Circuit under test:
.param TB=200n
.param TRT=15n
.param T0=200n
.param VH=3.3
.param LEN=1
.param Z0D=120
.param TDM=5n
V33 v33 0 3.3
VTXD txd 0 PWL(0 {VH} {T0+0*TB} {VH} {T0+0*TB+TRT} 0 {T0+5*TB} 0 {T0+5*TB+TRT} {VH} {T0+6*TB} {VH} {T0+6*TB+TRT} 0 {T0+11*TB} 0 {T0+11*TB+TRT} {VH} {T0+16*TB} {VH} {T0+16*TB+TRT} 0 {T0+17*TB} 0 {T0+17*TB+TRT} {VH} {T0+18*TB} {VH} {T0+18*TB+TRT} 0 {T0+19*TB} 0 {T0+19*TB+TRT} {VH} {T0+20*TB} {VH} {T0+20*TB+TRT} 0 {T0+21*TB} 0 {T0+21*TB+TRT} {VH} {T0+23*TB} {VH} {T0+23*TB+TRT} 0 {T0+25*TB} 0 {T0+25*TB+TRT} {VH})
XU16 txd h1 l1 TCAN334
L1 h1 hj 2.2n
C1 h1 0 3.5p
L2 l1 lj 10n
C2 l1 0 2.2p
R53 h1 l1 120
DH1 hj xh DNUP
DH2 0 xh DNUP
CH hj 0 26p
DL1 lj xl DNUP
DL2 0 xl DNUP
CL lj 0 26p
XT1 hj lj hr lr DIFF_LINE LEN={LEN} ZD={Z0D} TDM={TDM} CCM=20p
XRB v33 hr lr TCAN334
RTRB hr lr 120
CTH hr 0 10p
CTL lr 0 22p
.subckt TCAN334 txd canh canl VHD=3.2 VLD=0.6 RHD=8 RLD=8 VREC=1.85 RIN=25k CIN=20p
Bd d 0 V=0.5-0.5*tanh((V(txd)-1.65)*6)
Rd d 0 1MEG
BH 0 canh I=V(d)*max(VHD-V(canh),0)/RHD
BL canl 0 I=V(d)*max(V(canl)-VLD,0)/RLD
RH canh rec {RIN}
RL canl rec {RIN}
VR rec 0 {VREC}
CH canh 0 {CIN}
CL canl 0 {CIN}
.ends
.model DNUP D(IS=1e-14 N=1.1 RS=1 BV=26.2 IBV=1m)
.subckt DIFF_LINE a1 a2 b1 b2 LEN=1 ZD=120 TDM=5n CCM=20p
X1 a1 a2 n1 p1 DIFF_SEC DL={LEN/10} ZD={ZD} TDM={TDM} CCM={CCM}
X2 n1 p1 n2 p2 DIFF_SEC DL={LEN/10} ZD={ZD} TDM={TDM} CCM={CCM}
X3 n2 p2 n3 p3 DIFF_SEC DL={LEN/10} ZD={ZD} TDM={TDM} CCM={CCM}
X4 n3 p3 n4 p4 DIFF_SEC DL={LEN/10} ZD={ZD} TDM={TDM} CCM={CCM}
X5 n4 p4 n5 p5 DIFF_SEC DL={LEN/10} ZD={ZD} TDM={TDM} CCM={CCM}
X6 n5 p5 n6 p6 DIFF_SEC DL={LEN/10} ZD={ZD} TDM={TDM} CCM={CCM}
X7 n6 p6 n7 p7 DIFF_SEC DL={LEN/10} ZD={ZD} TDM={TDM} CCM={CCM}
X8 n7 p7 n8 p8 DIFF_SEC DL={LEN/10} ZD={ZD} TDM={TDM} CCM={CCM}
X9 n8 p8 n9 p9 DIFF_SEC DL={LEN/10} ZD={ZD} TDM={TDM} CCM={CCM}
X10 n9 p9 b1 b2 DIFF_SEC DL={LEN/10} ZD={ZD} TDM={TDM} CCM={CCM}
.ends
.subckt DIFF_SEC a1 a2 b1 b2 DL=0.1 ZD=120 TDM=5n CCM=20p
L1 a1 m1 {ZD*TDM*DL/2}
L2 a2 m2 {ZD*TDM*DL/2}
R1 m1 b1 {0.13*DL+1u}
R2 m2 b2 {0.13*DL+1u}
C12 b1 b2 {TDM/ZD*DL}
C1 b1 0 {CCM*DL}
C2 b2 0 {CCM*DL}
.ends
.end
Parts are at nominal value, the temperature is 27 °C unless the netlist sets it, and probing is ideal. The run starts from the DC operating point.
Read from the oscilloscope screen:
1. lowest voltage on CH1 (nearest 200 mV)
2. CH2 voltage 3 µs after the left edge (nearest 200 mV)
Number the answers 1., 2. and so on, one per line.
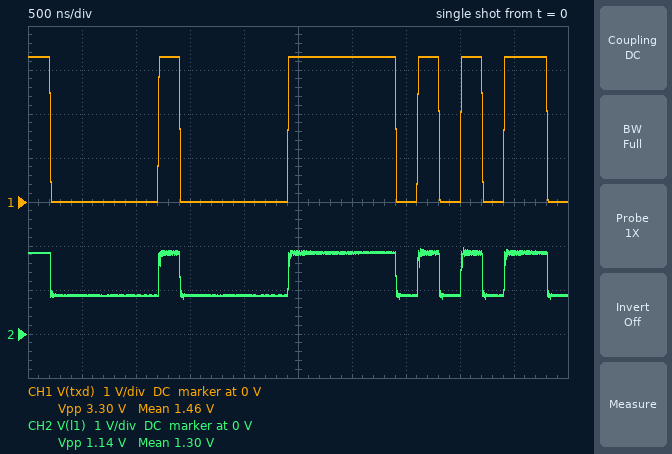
1. 0 V
2. 1.8 V
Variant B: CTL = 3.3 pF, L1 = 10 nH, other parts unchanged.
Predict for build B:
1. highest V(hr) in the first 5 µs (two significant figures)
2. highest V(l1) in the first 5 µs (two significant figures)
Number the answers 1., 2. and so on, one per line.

1. 3.2 V
2. 2.0 V
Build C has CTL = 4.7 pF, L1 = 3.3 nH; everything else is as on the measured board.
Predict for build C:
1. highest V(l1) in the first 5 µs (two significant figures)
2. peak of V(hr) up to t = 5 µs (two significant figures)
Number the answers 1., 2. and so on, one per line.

1. 2.0 V
2. 3.2 V
